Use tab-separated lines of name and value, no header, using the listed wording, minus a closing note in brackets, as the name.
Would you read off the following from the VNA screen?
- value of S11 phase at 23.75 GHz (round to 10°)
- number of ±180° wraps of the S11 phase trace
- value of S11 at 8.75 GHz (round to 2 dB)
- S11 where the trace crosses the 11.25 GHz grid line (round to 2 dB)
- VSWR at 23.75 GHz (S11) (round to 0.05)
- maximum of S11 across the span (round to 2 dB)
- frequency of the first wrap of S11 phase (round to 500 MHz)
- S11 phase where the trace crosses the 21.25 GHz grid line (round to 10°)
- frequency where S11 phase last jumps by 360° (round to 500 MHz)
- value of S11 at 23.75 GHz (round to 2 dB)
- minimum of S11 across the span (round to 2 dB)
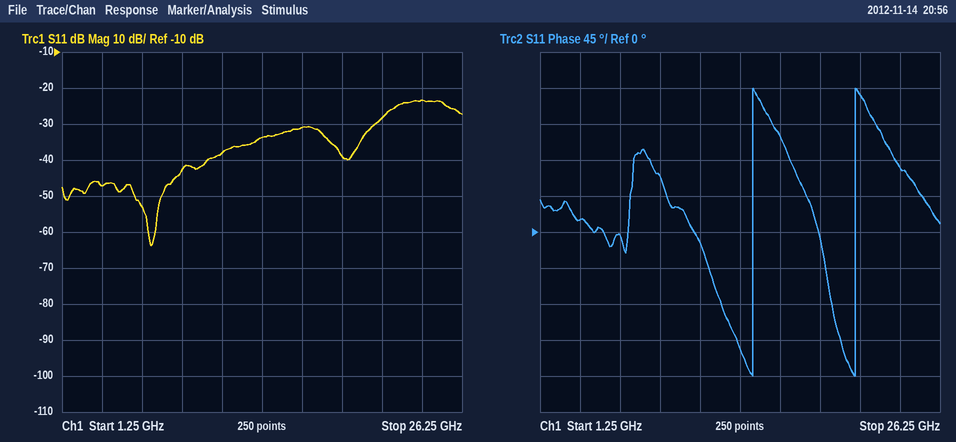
value of S11 phase at 23.75 GHz	80°
number of ±180° wraps of the S11 phase trace	2
value of S11 at 8.75 GHz	-42 dB
S11 where the trace crosses the 11.25 GHz grid line	-38 dB
VSWR at 23.75 GHz (S11)	1.15
maximum of S11 across the span	-24 dB
frequency of the first wrap of S11 phase	14.5 GHz
S11 phase where the trace crosses the 21.25 GHz grid line	170°
frequency where S11 phase last jumps by 360°	21.0 GHz
value of S11 at 23.75 GHz	-24 dB
minimum of S11 across the span	-64 dB
